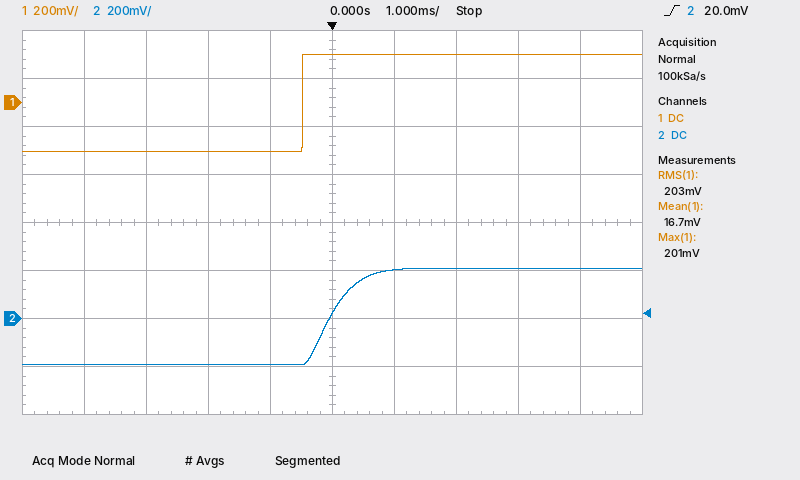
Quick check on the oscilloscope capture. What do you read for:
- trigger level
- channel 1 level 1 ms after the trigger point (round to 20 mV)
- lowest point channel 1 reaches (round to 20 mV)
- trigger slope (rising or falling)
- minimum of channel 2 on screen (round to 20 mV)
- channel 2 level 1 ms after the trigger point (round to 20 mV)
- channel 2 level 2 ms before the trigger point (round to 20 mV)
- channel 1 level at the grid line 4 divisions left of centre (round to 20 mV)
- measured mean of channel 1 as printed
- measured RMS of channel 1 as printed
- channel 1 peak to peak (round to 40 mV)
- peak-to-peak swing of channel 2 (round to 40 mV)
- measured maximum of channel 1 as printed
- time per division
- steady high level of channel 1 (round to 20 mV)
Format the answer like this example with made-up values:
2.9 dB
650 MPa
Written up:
20.0 mV
200 mV
-200 mV
rising
-200 mV
200 mV
-200 mV
-200 mV
16.7 mV
203 mV
400 mV
400 mV
201 mV
1 ms
200 mV
